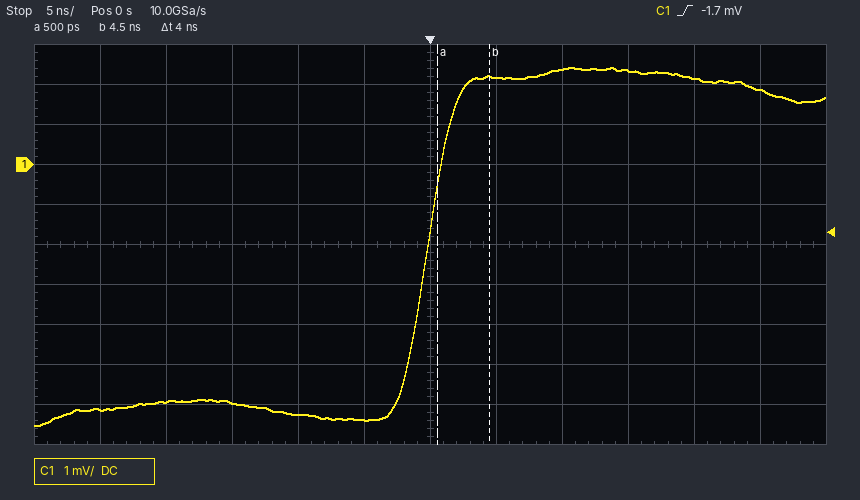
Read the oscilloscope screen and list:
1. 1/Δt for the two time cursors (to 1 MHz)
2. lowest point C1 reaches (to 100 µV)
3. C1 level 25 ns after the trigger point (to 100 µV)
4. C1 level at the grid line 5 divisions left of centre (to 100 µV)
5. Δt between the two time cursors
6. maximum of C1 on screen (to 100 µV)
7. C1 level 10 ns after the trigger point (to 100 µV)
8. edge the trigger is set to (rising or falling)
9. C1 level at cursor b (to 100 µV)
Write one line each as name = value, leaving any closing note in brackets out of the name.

1/Δt for the two time cursors = 250 MHz
lowest point C1 reaches = -6.5 mV
C1 level 25 ns after the trigger point = 1.9 mV
C1 level at the grid line 5 divisions left of centre = -6.1 mV
Δt between the two time cursors = 4 ns
maximum of C1 on screen = 2.4 mV
C1 level 10 ns after the trigger point = 2.4 mV
edge the trigger is set to = rising
C1 level at cursor b = 2.2 mV
